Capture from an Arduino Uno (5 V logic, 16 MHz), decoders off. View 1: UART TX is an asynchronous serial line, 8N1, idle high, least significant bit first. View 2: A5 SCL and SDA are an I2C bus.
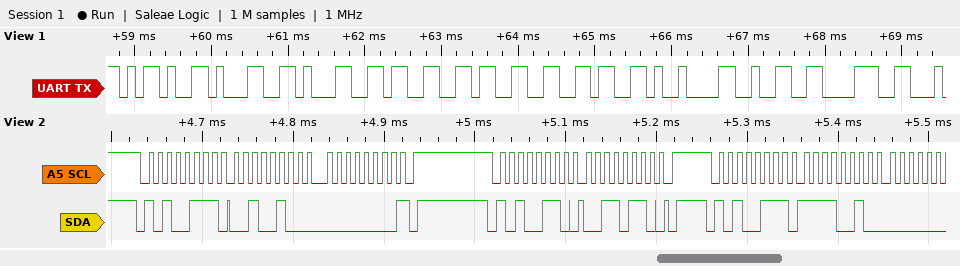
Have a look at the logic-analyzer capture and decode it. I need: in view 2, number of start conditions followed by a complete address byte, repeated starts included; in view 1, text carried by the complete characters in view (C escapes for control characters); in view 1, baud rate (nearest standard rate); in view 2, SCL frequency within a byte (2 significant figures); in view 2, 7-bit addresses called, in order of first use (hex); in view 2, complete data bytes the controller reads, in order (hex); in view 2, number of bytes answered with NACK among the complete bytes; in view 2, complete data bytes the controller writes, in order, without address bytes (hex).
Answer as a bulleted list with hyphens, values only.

- 3
- "-11336\t28"
- 9600 baud
- 100 kHz
- 0x53
- 24 00 F2
- 1
- 36
